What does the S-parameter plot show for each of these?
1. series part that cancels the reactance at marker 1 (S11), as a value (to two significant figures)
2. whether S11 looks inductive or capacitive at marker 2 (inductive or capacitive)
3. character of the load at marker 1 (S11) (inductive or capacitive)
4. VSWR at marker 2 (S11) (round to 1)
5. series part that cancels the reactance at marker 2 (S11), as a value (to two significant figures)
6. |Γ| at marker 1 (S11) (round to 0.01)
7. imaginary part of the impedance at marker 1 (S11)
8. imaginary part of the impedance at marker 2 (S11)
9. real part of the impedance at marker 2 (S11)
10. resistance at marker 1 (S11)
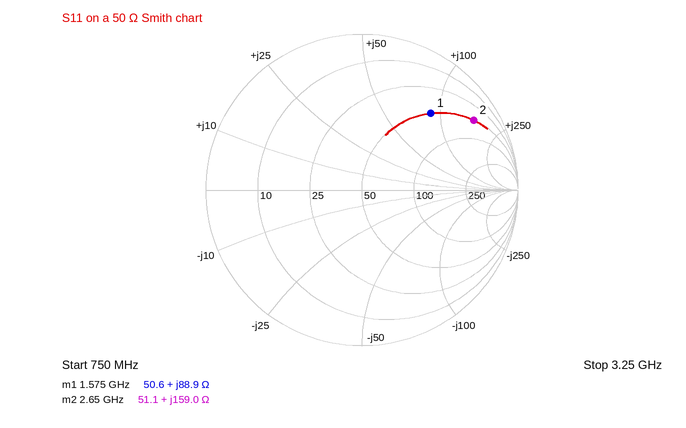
1.1 pF
inductive
inductive
12
380 fF
0.66
+88.9 Ω
+159.0 Ω
51.1 Ω
50.6 Ω
